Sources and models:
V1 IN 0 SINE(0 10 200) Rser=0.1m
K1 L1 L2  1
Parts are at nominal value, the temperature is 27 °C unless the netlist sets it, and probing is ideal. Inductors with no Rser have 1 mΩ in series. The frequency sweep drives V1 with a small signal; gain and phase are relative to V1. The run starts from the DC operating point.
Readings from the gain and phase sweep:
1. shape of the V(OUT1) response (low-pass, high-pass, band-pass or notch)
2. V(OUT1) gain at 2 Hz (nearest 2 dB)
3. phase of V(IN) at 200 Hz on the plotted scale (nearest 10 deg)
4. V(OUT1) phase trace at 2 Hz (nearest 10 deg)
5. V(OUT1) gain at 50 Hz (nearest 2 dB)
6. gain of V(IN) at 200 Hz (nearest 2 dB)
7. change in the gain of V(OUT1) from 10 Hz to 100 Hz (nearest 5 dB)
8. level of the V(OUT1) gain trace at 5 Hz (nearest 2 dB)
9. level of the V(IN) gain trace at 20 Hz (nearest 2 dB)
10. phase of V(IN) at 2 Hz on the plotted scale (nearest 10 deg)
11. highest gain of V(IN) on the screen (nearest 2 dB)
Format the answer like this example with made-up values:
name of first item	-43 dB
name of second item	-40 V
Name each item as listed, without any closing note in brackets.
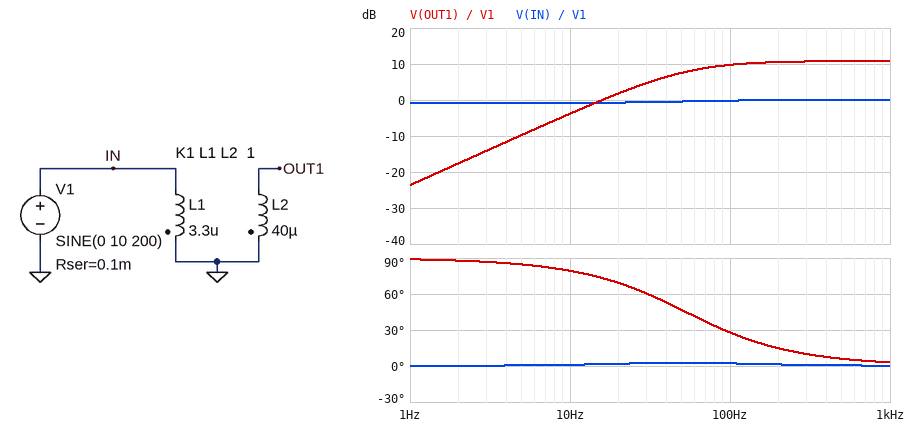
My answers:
shape of the V(OUT1) response	high-pass
V(OUT1) gain at 2 Hz	-18 dB
phase of V(IN) at 200 Hz on the plotted scale	0 deg
V(OUT1) phase trace at 2 Hz	90 deg
V(OUT1) gain at 50 Hz	8 dB
gain of V(IN) at 200 Hz	0 dB
change in the gain of V(OUT1) from 10 Hz to 100 Hz	15 dB
level of the V(OUT1) gain trace at 5 Hz	-10 dB
level of the V(IN) gain trace at 20 Hz	0 dB
phase of V(IN) at 2 Hz on the plotted scale	0 deg
highest gain of V(IN) on the screen	0 dB
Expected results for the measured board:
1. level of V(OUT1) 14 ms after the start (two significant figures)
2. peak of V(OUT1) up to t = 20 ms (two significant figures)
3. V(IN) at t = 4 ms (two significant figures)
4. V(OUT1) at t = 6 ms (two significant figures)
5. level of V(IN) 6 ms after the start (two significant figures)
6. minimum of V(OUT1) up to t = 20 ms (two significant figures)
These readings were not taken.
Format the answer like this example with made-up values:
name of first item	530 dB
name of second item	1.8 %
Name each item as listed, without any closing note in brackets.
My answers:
level of V(OUT1) 14 ms after the start	-28 V
peak of V(OUT1) up to t = 20 ms	34 V
V(IN) at t = 4 ms	-9.4 V
V(OUT1) at t = 6 ms	32 V
level of V(IN) 6 ms after the start	9.5 V
minimum of V(OUT1) up to t = 20 ms	-36 V
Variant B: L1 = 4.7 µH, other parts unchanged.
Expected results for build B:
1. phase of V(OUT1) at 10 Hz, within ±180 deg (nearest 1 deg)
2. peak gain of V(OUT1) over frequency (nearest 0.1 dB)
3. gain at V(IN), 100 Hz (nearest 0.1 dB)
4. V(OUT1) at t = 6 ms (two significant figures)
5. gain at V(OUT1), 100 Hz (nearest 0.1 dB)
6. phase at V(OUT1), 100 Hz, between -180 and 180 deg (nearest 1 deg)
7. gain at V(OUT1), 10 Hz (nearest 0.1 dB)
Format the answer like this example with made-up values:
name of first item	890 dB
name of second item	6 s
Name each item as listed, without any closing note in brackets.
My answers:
phase of V(OUT1) at 10 Hz, within ±180 deg	75 deg
peak gain of V(OUT1) over frequency	9.3 dB
gain at V(IN), 100 Hz	-0.1 dB
V(OUT1) at t = 6 ms	27 V
gain at V(OUT1), 100 Hz	8.7 dB
phase at V(OUT1), 100 Hz, between -180 and 180 deg	20 deg
gain at V(OUT1), 10 Hz	-2.4 dB
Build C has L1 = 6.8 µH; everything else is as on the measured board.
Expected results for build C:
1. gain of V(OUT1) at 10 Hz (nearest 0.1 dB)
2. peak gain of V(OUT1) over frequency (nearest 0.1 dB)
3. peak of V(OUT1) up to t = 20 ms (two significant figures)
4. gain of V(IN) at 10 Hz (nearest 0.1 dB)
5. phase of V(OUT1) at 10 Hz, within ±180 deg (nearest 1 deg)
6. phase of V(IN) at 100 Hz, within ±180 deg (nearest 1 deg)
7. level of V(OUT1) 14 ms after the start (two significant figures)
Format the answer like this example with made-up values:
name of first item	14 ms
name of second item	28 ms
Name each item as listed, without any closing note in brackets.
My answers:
gain of V(OUT1) at 10 Hz	-1.1 dB
peak gain of V(OUT1) over frequency	7.7 dB
peak of V(OUT1) up to t = 20 ms	24 V
gain of V(IN) at 10 Hz	-0.7 dB
phase of V(OUT1) at 10 Hz, within ±180 deg	69 deg
phase of V(IN) at 100 Hz, within ±180 deg	1 deg
level of V(OUT1) 14 ms after the start	-22 V
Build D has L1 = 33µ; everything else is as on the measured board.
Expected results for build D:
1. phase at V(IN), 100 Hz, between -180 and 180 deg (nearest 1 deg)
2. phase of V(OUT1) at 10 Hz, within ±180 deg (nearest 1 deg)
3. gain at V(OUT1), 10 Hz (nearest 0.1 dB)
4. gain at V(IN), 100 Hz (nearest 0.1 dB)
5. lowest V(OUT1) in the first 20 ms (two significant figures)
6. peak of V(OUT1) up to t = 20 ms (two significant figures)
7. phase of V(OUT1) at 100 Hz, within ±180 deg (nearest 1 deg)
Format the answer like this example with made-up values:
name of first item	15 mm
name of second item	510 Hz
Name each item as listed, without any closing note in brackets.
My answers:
phase at V(IN), 100 Hz, between -180 and 180 deg	0 deg
phase of V(OUT1) at 10 Hz, within ±180 deg	28 deg
gain at V(OUT1), 10 Hz	-0.2 dB
gain at V(IN), 100 Hz	0 dB
lowest V(OUT1) in the first 20 ms	-11 V
peak of V(OUT1) up to t = 20 ms	11 V
phase of V(OUT1) at 100 Hz, within ±180 deg	3 deg
